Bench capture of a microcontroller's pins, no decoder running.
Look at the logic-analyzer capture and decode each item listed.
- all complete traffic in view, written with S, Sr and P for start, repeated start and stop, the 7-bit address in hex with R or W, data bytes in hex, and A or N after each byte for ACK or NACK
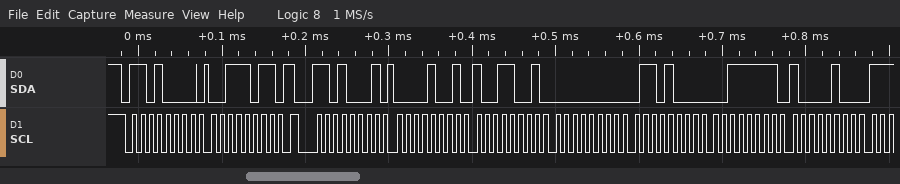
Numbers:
S 68W A 3B A Sr 68R A 09 A 99 A 00 A 68 A 3F A 84 A
